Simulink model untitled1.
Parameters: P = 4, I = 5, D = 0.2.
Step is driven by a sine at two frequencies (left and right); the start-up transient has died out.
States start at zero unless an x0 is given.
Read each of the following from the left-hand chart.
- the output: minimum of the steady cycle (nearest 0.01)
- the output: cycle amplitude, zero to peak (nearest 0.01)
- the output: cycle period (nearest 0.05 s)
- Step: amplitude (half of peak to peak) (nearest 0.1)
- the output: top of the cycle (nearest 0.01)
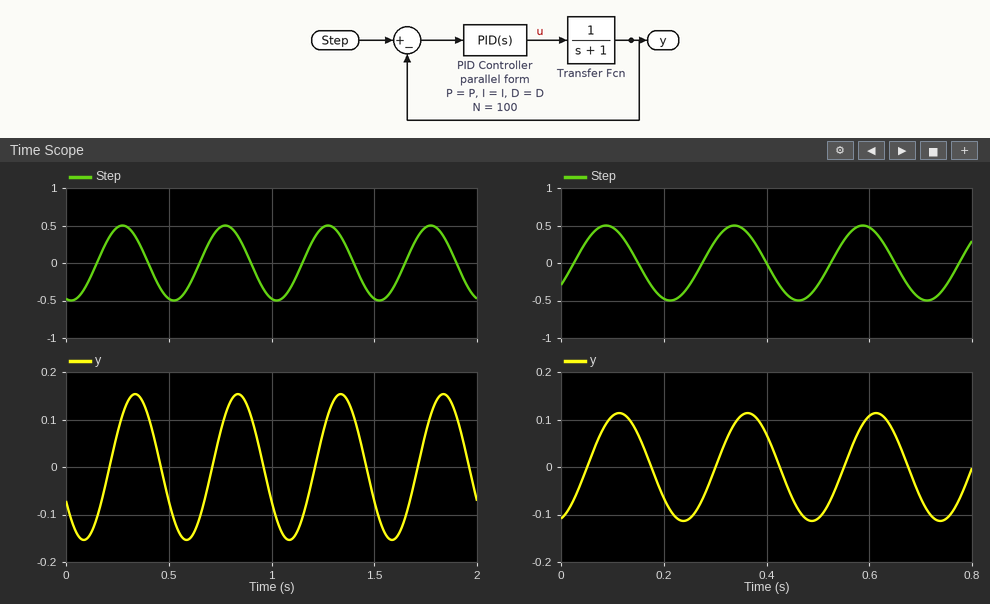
-0.15
0.15
0.50 s
0.5
0.15
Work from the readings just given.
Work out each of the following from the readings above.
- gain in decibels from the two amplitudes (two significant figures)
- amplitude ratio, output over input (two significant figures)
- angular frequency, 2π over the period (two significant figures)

-10 dB
0.30
13 rad/s
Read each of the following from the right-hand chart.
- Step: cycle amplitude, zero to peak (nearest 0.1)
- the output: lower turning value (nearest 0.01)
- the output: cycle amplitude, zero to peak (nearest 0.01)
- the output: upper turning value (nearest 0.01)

0.5
-0.11
0.11
0.11
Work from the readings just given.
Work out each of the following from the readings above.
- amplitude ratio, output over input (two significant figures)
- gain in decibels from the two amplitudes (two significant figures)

0.22
-13 dB
